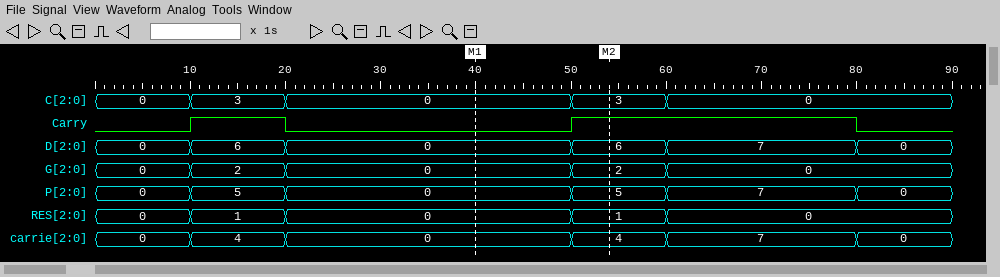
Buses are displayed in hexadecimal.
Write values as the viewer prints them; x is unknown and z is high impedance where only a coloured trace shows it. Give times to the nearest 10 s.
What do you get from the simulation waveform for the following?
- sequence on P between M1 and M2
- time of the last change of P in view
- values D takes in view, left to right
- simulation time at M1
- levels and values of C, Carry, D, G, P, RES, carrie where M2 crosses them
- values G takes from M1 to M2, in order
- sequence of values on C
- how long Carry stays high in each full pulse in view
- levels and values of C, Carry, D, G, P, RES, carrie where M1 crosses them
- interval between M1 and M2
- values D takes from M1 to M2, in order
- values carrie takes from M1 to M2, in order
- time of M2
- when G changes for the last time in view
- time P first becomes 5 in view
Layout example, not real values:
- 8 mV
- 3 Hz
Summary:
- 0, 5
- 80 s
- 0, 6, 0, 6, 7, 0
- 40 s
- C=3, Carry=1, D=6, G=2, P=5, RES=1, carrie=4
- 0, 2
- 0, 3, 0, 3, 0
- 10 s, 30 s
- C=0, Carry=0, D=0, G=0, P=0, RES=0, carrie=0
- 10 s
- 0, 6
- 0, 4
- 50 s
- 60 s
- 10 s
